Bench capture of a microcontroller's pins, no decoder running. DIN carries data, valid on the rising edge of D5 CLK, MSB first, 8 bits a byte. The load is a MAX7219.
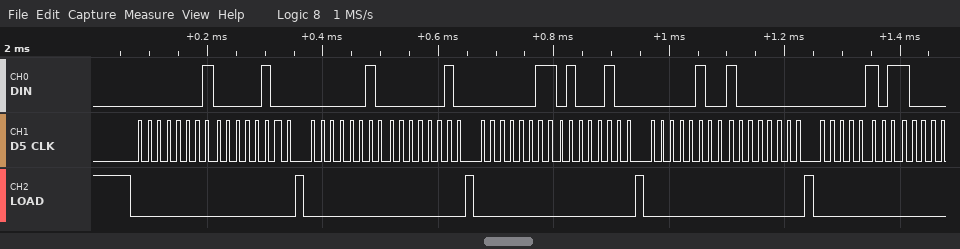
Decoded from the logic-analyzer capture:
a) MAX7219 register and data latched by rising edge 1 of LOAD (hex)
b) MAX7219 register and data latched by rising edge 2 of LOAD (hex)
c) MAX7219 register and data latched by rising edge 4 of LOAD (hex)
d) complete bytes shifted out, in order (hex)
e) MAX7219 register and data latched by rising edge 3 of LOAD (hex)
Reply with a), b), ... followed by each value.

a) register 0x1, data 0x04
b) register 0x2, data 0x02
c) register 0x4, data 0x80
d) 01 04 02 02 03 44 04 80 05
e) register 0x3, data 0x44
